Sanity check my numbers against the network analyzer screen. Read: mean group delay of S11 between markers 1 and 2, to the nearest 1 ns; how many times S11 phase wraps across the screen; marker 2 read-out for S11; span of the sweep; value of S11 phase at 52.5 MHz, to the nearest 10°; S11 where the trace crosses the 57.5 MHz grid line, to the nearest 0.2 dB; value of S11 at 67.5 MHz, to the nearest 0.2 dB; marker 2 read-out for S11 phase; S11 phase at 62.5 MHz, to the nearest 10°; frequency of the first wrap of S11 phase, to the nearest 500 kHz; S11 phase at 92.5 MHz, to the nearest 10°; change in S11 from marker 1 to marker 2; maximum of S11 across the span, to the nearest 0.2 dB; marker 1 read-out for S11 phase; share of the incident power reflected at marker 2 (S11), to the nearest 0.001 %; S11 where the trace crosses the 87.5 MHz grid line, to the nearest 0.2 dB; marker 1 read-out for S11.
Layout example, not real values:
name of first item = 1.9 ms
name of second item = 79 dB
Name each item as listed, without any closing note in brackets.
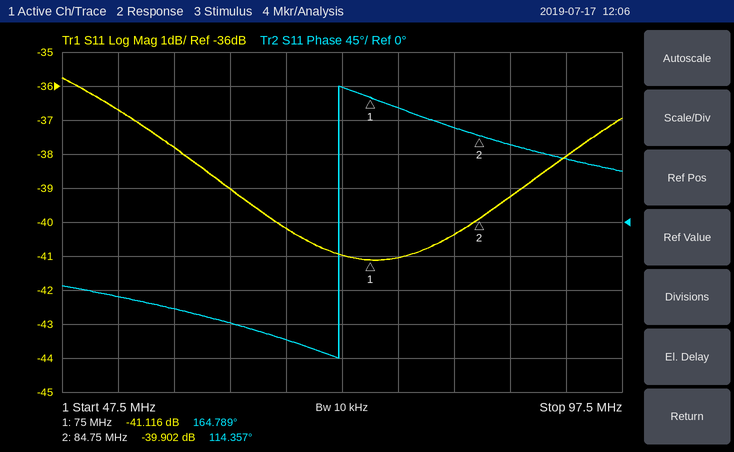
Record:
mean group delay of S11 between markers 1 and 2, to the nearest 1 ns = 14 ns
how many times S11 phase wraps across the screen = 1
marker 2 read-out for S11 = -39.902 dB
span of the sweep = 50 MHz
value of S11 phase at 52.5 MHz, to the nearest 10° = -100°
S11 where the trace crosses the 57.5 MHz grid line, to the nearest 0.2 dB = -37.8 dB
value of S11 at 67.5 MHz, to the nearest 0.2 dB = -40.2 dB
marker 2 read-out for S11 phase = 114.357°
S11 phase at 62.5 MHz, to the nearest 10° = -130°
frequency of the first wrap of S11 phase, to the nearest 500 kHz = 72.0 MHz
S11 phase at 92.5 MHz, to the nearest 10° = 80°
change in S11 from marker 1 to marker 2 = 1.214 dB
maximum of S11 across the span, to the nearest 0.2 dB = -35.8 dB
marker 1 read-out for S11 phase = 164.789°
share of the incident power reflected at marker 2 (S11), to the nearest 0.001 % = 0.010 %
S11 where the trace crosses the 87.5 MHz grid line, to the nearest 0.2 dB = -39.2 dB
marker 1 read-out for S11 = -41.116 dB
